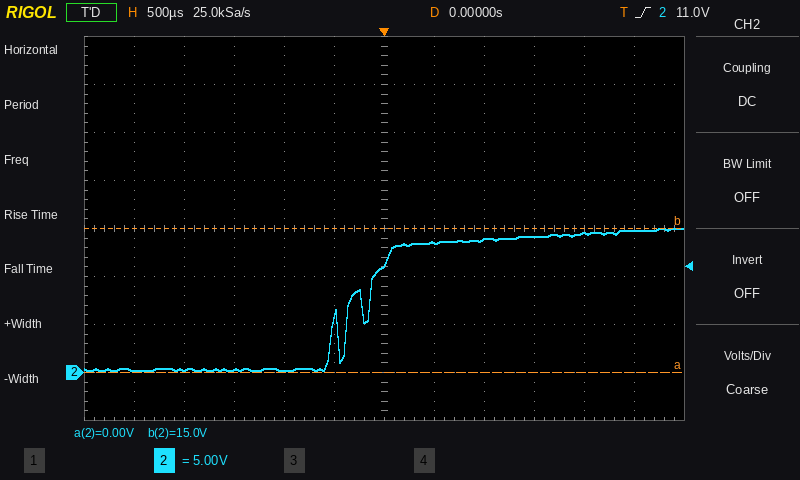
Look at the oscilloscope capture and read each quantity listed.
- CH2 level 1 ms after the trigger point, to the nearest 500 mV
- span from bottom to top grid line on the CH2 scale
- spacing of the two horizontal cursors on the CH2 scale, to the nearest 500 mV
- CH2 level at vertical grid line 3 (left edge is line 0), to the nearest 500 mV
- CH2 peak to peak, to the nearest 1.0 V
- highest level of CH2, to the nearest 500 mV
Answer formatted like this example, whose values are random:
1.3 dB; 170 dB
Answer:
14.0 V; 40 V; 15.0 V; 500 mV; 15.0 V; 15.0 V
